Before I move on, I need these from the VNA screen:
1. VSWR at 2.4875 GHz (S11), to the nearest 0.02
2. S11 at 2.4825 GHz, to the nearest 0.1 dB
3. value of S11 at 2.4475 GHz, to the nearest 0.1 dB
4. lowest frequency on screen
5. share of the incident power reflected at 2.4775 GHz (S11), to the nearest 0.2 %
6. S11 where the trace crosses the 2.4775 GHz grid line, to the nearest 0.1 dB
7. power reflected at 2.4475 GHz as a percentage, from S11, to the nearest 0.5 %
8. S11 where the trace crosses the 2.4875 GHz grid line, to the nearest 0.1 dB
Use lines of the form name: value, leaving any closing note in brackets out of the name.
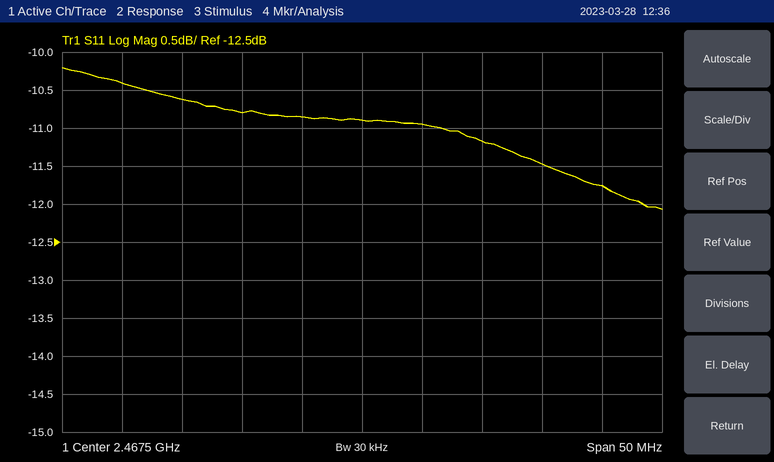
VSWR at 2.4875 GHz (S11), to the nearest 0.02: 1.70
S11 at 2.4825 GHz, to the nearest 0.1 dB: -11.5 dB
value of S11 at 2.4475 GHz, to the nearest 0.1 dB: -10.4 dB
lowest frequency on screen: 2.4425 GHz
share of the incident power reflected at 2.4775 GHz (S11), to the nearest 0.2 %: 7.6 %
S11 where the trace crosses the 2.4775 GHz grid line, to the nearest 0.1 dB: -11.2 dB
power reflected at 2.4475 GHz as a percentage, from S11, to the nearest 0.5 %: 9.0 %
S11 where the trace crosses the 2.4875 GHz grid line, to the nearest 0.1 dB: -11.8 dB
